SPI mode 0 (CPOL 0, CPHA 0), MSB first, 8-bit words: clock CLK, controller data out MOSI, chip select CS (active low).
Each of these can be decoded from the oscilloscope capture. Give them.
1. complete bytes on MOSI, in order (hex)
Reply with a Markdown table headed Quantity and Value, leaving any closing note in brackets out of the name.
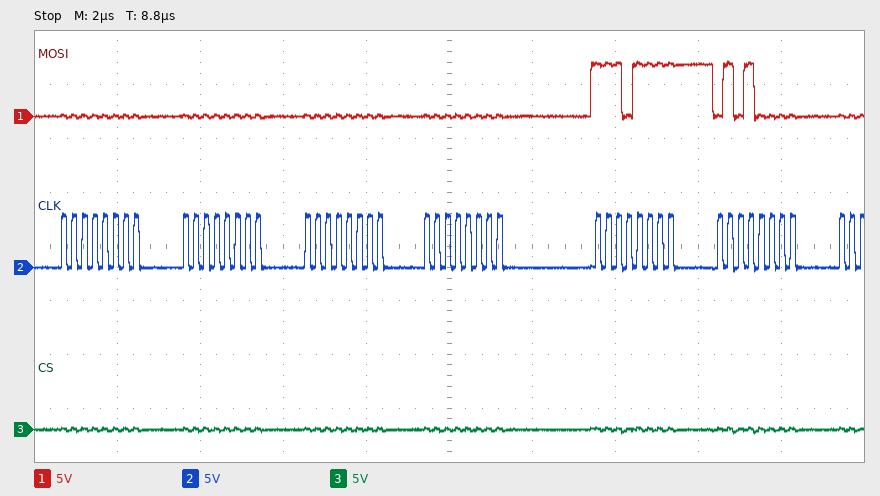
| Quantity | Value |
|---|---|
| complete bytes on MOSI, in order | 00 00 00 00 EF 50 |
